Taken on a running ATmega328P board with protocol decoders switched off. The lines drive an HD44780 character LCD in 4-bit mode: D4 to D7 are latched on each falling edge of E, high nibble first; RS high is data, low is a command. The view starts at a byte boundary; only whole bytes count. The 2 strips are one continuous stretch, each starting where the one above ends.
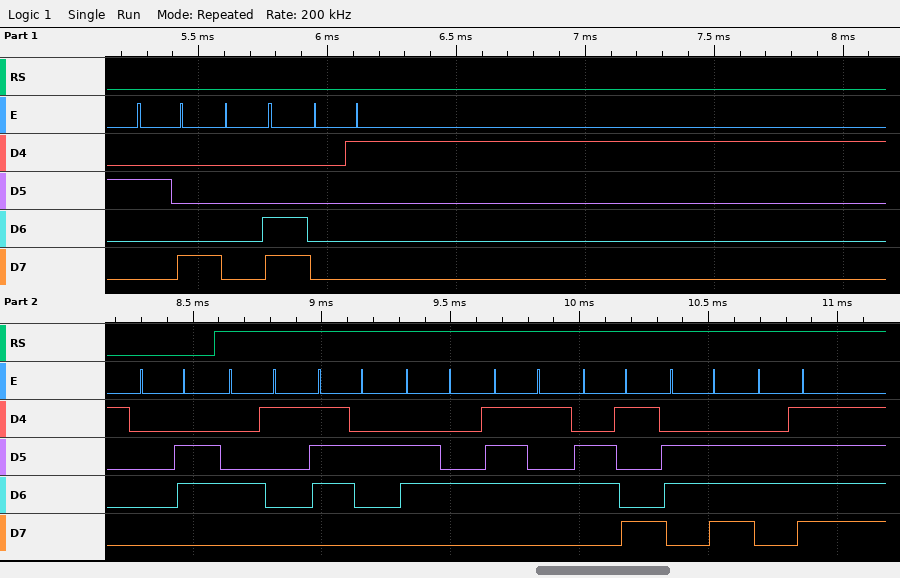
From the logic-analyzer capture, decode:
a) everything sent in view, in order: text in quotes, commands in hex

0x28 0x0C 0x01 0x06 "Arduino"
